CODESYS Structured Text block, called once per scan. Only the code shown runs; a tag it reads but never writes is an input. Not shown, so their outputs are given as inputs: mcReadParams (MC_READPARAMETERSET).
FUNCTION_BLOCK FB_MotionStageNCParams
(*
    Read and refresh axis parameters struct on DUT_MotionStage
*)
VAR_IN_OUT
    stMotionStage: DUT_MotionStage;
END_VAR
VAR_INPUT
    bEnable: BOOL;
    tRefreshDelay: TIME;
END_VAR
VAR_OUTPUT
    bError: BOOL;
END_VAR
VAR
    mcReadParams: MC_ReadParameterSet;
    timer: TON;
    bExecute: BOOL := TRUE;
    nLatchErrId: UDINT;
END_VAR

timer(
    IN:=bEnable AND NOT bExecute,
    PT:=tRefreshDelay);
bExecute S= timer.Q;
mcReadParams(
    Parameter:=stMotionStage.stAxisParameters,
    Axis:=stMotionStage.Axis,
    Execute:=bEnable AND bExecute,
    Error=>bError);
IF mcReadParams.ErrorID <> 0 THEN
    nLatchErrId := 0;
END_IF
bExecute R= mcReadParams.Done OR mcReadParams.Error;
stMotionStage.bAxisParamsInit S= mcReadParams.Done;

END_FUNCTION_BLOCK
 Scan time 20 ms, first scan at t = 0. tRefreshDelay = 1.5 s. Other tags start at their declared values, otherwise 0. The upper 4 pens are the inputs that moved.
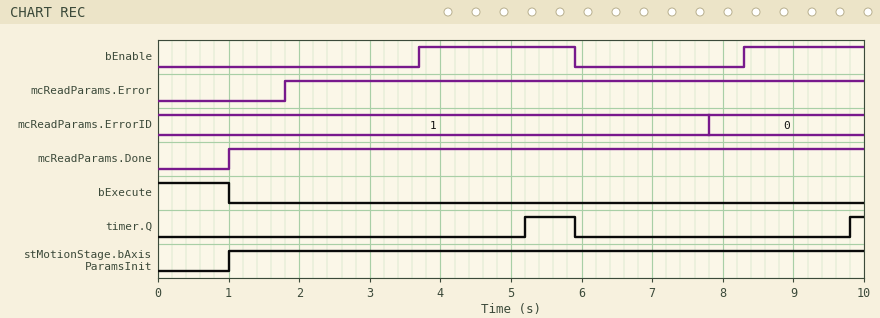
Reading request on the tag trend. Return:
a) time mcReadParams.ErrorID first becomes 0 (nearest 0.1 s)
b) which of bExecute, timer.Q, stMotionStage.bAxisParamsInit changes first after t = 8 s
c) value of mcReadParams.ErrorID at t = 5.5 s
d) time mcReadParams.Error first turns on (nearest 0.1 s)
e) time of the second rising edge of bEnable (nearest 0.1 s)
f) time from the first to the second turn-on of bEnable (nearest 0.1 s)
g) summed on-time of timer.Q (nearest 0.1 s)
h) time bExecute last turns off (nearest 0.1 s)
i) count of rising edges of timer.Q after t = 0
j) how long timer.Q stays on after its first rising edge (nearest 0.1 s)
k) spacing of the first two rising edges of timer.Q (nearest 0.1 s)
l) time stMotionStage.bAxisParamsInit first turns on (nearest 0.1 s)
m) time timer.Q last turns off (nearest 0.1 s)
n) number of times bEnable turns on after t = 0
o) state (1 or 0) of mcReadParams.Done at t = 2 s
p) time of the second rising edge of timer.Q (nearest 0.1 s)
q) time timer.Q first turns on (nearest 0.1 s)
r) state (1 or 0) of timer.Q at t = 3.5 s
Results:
7.8 s
timer.Q
1
1.8 s
8.3 s
4.6 s
0.9 s
1.0 s
2
0.7 s
4.6 s
1.0 s
5.9 s
2
1
9.8 s
5.2 s
0
